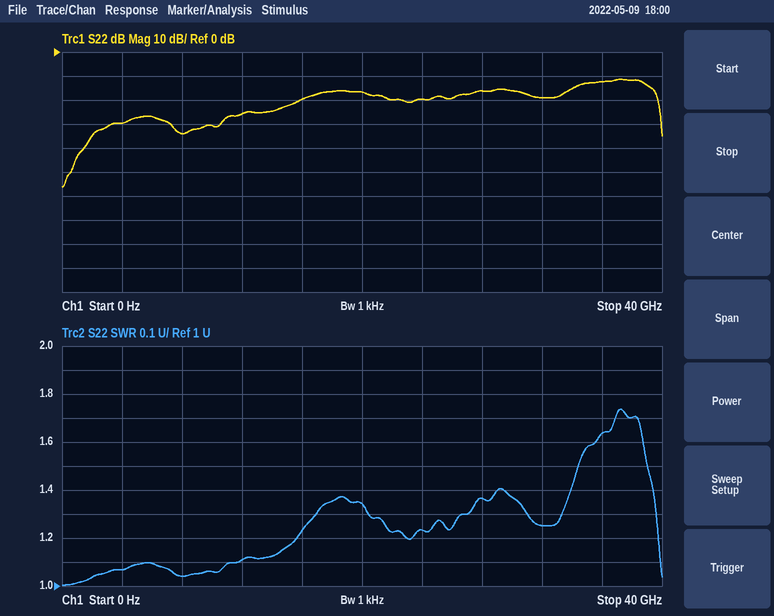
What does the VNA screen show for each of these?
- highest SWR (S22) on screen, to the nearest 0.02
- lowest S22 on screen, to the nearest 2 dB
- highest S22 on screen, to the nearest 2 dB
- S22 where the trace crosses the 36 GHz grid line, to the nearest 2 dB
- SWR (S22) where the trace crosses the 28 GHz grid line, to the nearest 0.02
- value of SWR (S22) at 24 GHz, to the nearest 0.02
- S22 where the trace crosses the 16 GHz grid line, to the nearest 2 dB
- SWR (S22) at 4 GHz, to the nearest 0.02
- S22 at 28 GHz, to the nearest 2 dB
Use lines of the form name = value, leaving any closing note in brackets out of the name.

highest SWR (S22) on screen, to the nearest 0.02 = 1.74
lowest S22 on screen, to the nearest 2 dB = -56 dB
highest S22 on screen, to the nearest 2 dB = -12 dB
S22 where the trace crosses the 36 GHz grid line, to the nearest 2 dB = -12 dB
SWR (S22) where the trace crosses the 28 GHz grid line, to the nearest 0.02 = 1.36
value of SWR (S22) at 24 GHz, to the nearest 0.02 = 1.24
S22 where the trace crosses the 16 GHz grid line, to the nearest 2 dB = -20 dB
SWR (S22) at 4 GHz, to the nearest 0.02 = 1.06
S22 at 28 GHz, to the nearest 2 dB = -16 dB
